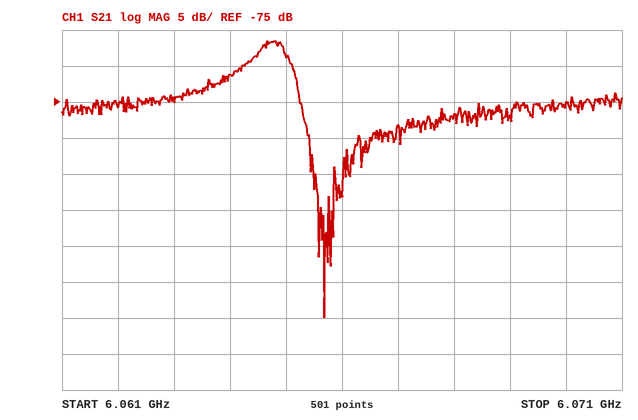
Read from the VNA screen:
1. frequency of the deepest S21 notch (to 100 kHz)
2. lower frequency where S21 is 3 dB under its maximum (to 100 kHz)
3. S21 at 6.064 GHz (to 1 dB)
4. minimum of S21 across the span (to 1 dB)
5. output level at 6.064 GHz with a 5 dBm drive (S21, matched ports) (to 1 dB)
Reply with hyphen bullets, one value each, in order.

- 6.0657 GHz
- 6.0643 GHz
- -71 dB
- -105 dB
- -66 dBm
